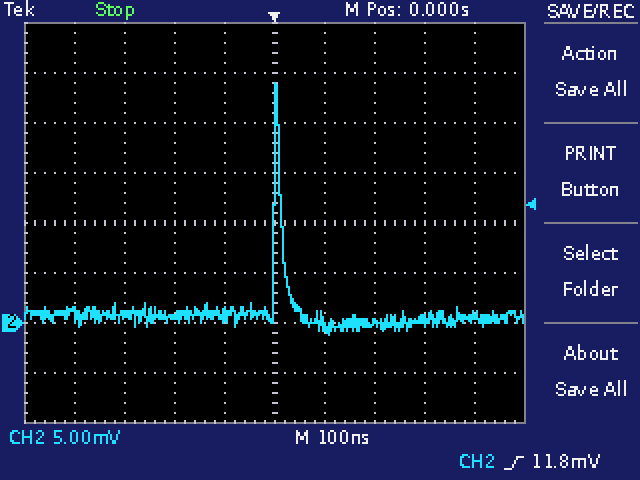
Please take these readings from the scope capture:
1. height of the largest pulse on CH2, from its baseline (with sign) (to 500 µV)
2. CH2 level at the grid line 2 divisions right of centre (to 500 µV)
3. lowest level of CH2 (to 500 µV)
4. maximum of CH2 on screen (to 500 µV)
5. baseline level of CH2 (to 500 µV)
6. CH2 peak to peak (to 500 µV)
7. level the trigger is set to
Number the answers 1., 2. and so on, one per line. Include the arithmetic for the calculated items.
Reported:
1. 24.0 mV − (500 µV) = +23.5 mV
2. 0.0 mV
3. -1.0 mV
4. 24.0 mV
5. 500 µV
6. 24.0 mV − (-1.0 mV) = 25.0 mV
7. 11.8 mV
